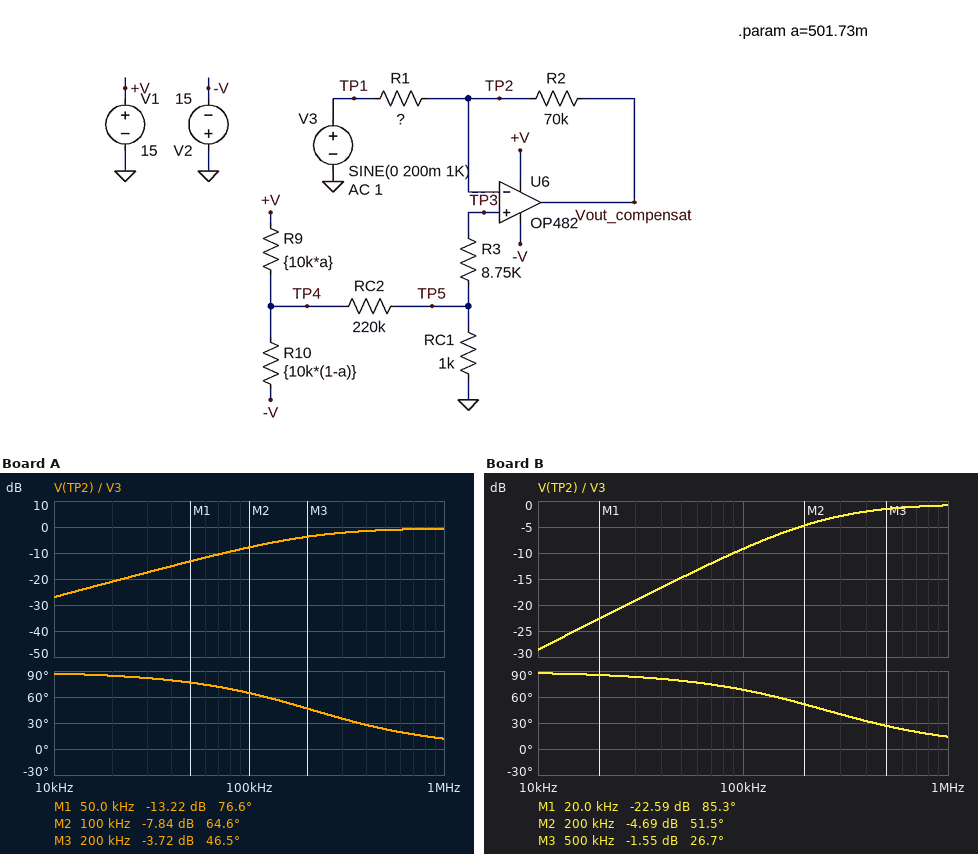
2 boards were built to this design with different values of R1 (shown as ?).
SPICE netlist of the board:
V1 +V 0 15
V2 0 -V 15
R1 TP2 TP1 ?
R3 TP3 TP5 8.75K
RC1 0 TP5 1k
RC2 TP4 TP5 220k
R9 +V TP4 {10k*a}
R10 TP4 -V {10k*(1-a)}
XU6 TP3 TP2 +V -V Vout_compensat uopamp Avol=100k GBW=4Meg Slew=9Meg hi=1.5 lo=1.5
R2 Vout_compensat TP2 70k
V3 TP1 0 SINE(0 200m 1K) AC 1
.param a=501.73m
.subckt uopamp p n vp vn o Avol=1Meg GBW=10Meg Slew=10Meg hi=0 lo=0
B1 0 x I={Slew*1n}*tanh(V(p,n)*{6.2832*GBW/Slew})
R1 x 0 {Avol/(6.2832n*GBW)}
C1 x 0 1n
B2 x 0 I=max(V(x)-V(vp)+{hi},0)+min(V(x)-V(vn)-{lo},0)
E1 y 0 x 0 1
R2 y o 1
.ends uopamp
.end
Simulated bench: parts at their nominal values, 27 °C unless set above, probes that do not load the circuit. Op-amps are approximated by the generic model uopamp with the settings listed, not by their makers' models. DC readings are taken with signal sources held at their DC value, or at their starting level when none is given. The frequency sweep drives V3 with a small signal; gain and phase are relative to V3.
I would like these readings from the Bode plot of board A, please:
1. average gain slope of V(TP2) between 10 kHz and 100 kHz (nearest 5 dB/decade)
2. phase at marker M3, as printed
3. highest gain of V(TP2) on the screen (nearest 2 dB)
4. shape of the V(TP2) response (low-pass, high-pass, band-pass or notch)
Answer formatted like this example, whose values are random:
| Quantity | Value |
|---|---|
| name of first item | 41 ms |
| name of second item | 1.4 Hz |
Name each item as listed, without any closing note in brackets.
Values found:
| Quantity | Value |
|---|---|
| average gain slope of V(TP2) between 10 kHz and 100 kHz | 20 dB/decade |
| phase at marker M3, as printed | 46.5 deg |
| highest gain of V(TP2) on the screen | 0 dB |
| shape of the V(TP2) response | high-pass |
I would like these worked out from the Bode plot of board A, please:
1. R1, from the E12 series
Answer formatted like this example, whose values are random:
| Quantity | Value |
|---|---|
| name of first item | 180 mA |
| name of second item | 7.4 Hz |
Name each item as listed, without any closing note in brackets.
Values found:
| Quantity | Value |
|---|---|
| R1, from the E12 series | 3.9 kΩ |
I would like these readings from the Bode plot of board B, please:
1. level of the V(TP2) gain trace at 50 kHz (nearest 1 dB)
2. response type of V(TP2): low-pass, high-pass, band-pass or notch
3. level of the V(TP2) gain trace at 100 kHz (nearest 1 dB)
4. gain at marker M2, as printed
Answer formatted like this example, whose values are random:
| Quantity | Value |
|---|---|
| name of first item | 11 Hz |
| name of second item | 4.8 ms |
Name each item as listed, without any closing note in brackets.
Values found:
| Quantity | Value |
|---|---|
| level of the V(TP2) gain trace at 50 kHz | -15 dB |
| response type of V(TP2): low-pass, high-pass, band-pass or notch | high-pass |
| level of the V(TP2) gain trace at 100 kHz | -9 dB |
| gain at marker M2, as printed | -4.69 dB |
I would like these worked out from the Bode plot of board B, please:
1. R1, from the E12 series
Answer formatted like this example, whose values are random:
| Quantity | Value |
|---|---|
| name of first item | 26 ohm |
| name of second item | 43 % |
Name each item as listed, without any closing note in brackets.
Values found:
| Quantity | Value |
|---|---|
| R1, from the E12 series | 4.7 kΩ |
